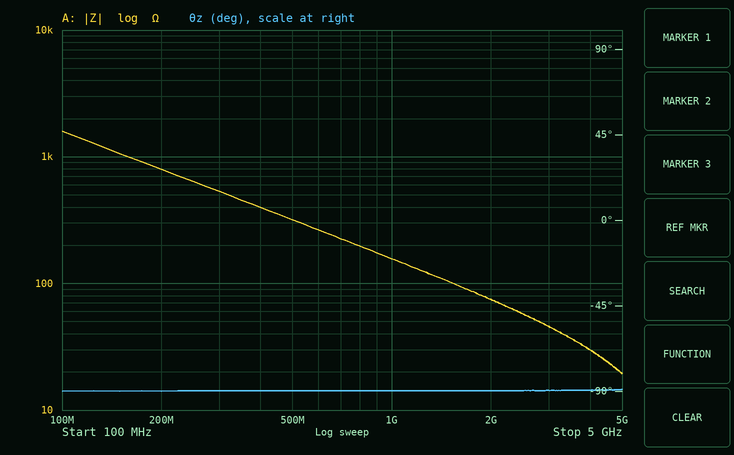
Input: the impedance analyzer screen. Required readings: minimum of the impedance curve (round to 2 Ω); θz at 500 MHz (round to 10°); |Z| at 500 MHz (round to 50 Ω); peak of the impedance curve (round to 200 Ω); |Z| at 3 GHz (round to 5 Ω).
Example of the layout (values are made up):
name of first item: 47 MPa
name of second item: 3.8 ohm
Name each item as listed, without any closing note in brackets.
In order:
minimum of the impedance curve: 20 Ω
θz at 500 MHz: -90°
|Z| at 500 MHz: 300 Ω
peak of the impedance curve: 1.6 kΩ
|Z| at 3 GHz: 45 Ω
